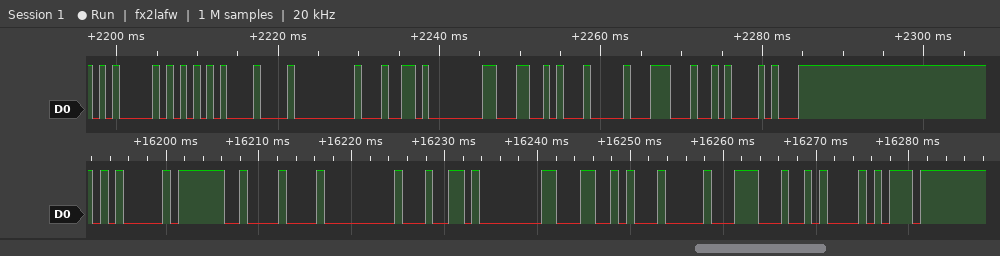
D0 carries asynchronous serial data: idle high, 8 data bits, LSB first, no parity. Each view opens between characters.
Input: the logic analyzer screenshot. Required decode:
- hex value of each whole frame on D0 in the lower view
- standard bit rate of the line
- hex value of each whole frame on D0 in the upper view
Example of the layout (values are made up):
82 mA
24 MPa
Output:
05, 3F, 08, 00, 64, 80, 4C, 04, 1C, 0A, DD
1200 baud
05, 55, 08, 00, 64, 80, 4C, 04, 1C, 0A, F1
